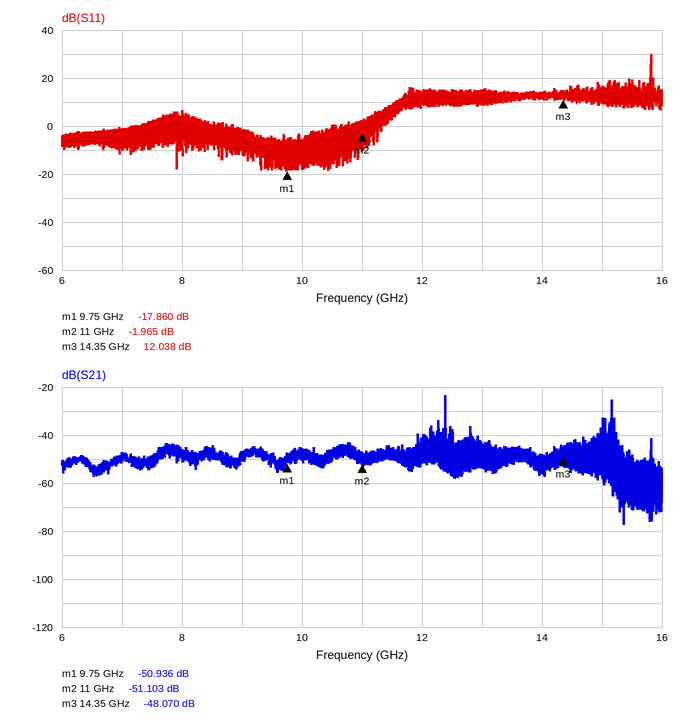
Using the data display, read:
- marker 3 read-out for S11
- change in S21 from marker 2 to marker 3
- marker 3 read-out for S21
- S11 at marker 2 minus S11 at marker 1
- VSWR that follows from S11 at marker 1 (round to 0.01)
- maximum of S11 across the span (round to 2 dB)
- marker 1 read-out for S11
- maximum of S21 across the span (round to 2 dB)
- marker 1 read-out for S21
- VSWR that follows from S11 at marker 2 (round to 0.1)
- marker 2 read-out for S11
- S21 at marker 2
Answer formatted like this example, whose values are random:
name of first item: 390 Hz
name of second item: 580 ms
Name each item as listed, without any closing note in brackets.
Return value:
marker 3 read-out for S11: 12.038 dB
change in S21 from marker 2 to marker 3: 3.033 dB
marker 3 read-out for S21: -48.070 dB
S11 at marker 2 minus S11 at marker 1: 15.895 dB
VSWR that follows from S11 at marker 1: 1.29
maximum of S11 across the span: 30 dB
marker 1 read-out for S11: -17.860 dB
maximum of S21 across the span: -24 dB
marker 1 read-out for S21: -50.936 dB
VSWR that follows from S11 at marker 2: 8.9
marker 2 read-out for S11: -1.965 dB
S21 at marker 2: -51.103 dB
